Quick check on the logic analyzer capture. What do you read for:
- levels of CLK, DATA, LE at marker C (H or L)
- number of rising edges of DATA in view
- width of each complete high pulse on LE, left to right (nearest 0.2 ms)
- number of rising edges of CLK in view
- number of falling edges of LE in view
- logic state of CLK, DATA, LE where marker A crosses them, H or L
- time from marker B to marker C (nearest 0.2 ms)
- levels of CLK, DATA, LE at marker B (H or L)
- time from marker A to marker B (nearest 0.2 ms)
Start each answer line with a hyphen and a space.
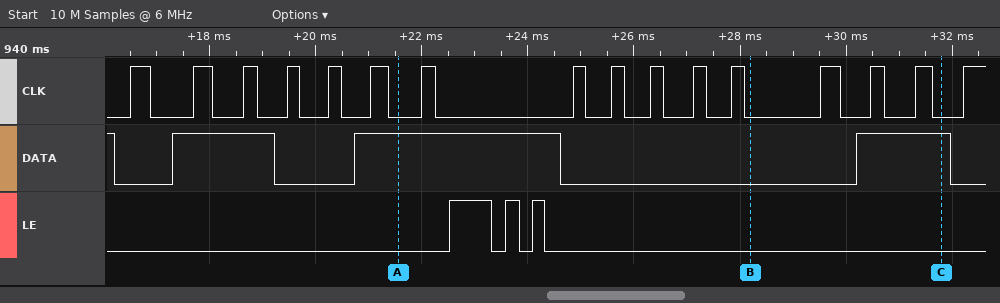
- CLK=L, DATA=H, LE=L
- 3
- 0.8 ms, 0.2 ms, 0.2 ms
- 16
- 3
- CLK=L, DATA=H, LE=L
- 3.6 ms
- CLK=L, DATA=L, LE=L
- 6.6 ms
